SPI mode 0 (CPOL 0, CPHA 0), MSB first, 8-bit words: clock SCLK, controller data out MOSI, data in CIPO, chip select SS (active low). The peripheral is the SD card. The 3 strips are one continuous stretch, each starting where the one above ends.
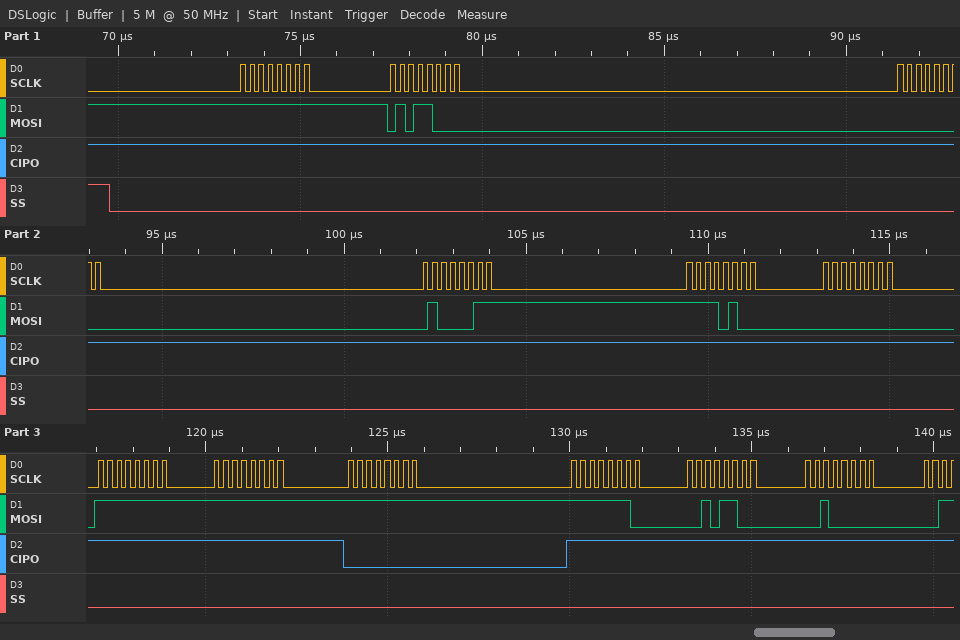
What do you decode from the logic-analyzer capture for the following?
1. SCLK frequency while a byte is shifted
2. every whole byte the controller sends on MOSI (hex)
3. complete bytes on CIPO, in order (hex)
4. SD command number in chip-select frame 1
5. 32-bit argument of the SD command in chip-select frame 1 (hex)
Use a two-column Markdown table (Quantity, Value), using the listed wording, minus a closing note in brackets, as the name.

| Quantity | Value |
|---|---|
| SCLK frequency while a byte is shifted | 4 MHz |
| every whole byte the controller sends on MOSI | 0xFF 0x58 0x00 0x43 0xF4 0x00 0xFF 0xFF 0xFF 0xFE 0x2C 0x20 |
| complete bytes on CIPO, in order | 0xFF 0xFF 0xFF 0xFF 0xFF 0xFF 0xFF 0xFF 0x00 0xFF 0xFF 0xFF |
| SD command number in chip-select frame 1 | CMD24 |
| 32-bit argument of the SD command in chip-select frame 1 | 0x0043F400 |
